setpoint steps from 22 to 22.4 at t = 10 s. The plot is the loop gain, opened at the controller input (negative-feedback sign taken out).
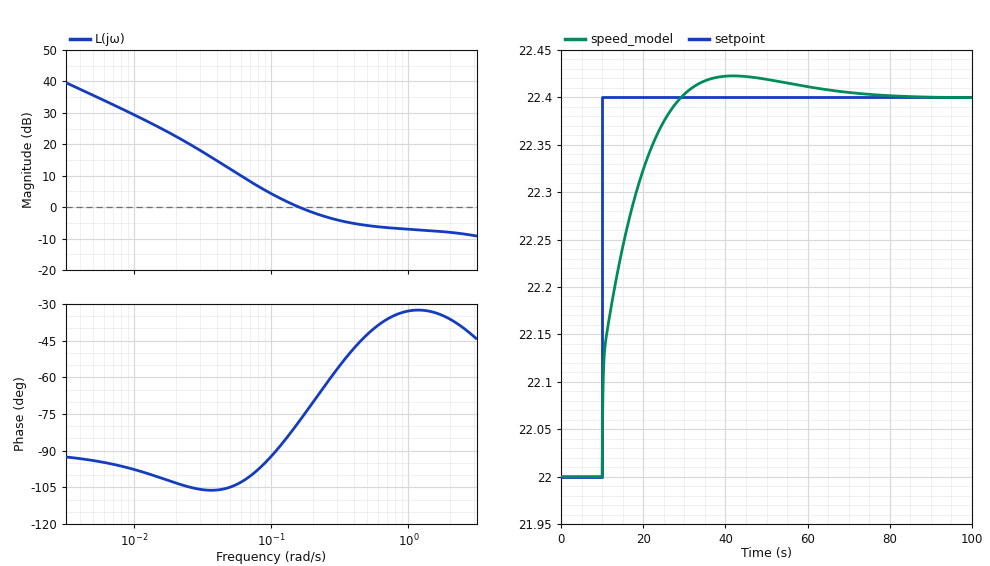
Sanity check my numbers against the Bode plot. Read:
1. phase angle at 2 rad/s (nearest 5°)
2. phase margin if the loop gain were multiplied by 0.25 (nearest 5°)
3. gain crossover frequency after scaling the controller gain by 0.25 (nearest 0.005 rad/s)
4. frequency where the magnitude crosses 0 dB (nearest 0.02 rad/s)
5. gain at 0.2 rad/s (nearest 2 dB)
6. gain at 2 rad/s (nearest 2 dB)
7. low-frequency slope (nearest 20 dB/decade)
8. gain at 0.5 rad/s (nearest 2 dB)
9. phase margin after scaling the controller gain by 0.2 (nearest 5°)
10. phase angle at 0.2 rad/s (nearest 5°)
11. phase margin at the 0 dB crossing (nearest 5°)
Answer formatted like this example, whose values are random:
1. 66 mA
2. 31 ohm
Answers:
1. -35°
2. 75°
3. 0.050 rad/s
4. 0.16 rad/s
5. -2 dB
6. -8 dB
7. -20 dB/decade
8. -6 dB
9. 75°
10. -70°
11. 100°
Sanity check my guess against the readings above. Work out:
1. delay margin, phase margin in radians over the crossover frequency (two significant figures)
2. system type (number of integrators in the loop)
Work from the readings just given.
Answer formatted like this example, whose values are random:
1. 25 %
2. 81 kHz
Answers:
1. 11 s
2. 1
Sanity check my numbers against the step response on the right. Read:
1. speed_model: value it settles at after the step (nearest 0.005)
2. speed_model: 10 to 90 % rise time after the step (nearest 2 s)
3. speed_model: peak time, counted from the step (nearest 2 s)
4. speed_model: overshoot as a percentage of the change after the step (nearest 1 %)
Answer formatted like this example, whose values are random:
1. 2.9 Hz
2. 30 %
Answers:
1. 22.400
2. 14 s
3. 32 s
4. 6 %
